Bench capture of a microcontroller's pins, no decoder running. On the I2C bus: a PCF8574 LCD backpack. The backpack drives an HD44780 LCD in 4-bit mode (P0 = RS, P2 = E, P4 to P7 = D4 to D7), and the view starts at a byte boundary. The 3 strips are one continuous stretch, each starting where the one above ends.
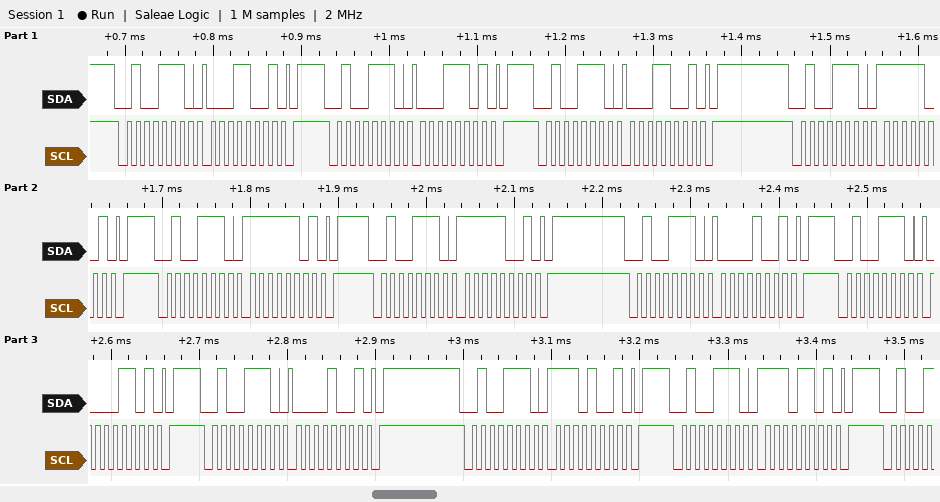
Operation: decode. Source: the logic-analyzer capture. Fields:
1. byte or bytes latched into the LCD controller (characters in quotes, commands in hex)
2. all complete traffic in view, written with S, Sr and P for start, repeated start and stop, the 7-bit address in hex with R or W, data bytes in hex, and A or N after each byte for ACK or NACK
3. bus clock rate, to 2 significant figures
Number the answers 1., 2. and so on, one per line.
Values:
1. data 0x1F
2. S 27W A 19 A P S 27W A 1D A P S 27W A 19 A P S 27W A F9 A P S 27W A FD A P S 27W A F9 A P S 27W A 09 A P S 27W A 0D A P S 27W A 09 A P S 27W A E9 A P S 27W A ED A P
3. 100 kHz
